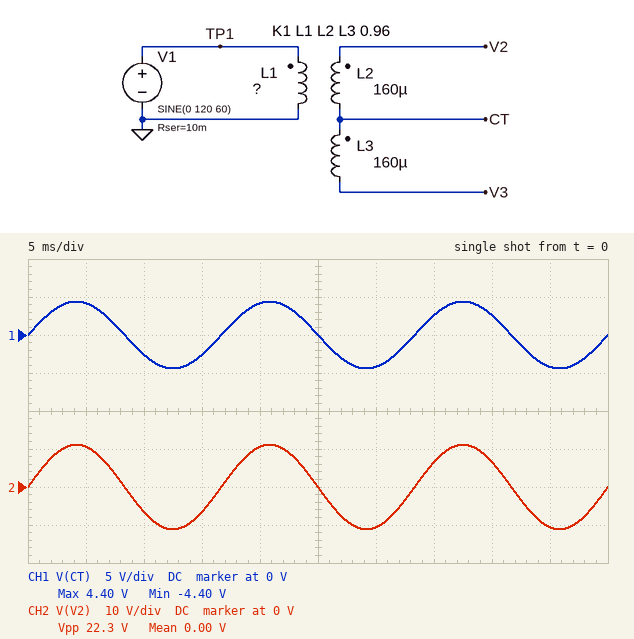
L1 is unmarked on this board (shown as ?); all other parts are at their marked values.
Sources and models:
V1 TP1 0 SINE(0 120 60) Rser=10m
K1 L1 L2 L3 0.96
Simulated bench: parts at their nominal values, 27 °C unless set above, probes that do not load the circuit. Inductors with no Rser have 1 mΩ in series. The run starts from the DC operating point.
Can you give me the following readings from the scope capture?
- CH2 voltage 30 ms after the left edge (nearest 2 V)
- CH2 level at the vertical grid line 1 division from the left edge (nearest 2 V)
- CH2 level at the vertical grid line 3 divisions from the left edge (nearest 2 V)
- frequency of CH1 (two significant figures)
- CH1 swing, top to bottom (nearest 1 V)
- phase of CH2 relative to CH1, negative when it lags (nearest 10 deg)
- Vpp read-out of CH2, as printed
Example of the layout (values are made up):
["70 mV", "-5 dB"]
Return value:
["-10 V", "10 V", "-6 V", "60 Hz", "9 V", "0 deg", "22.3 V"]
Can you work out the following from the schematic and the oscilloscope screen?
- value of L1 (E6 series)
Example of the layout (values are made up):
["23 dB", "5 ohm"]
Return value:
["47 mH"]
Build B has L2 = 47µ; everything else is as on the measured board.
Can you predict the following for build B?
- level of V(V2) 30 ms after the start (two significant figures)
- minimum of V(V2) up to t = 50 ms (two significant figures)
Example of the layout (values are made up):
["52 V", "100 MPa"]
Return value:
["-7.7 V", "-8.1 V"]
